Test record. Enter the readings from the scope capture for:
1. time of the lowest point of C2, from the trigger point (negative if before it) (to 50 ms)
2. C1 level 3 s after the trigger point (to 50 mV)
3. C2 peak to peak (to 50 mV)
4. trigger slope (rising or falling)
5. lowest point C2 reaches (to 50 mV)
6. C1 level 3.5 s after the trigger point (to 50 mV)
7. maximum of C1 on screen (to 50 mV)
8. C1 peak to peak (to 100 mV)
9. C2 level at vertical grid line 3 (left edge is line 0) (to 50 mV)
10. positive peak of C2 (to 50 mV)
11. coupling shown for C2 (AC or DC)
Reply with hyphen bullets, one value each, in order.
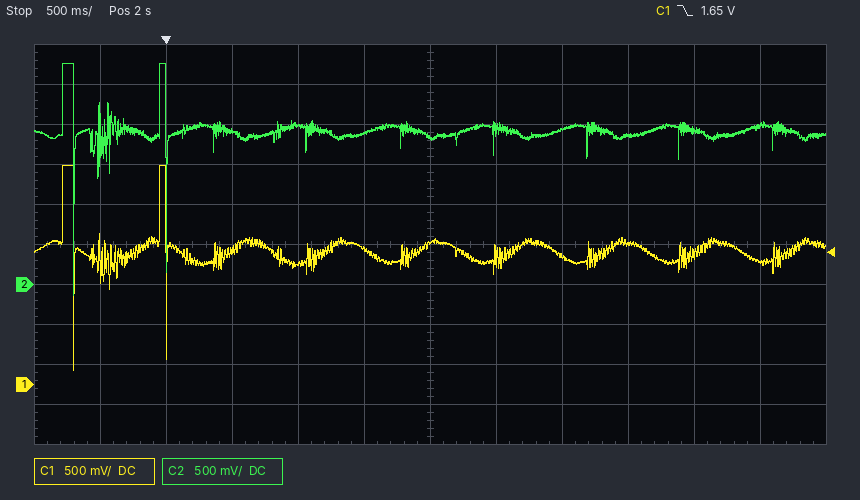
- -700 ms
- 1.60 V
- 2.90 V
- falling
- -150 mV
- 1.75 V
- 2.75 V
- 2.60 V
- 1.90 V
- 2.75 V
- DC
